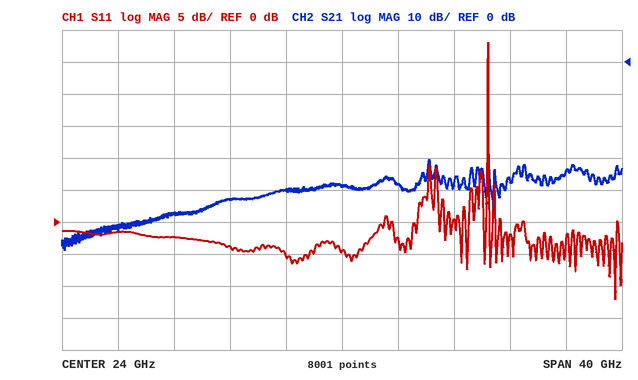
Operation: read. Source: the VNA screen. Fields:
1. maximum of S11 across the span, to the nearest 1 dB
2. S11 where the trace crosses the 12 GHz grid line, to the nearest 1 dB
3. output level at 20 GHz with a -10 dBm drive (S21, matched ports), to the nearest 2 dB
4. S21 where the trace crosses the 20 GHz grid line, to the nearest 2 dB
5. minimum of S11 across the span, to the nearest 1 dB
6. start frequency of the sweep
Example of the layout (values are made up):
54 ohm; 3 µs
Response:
28 dB; -2 dB; -50 dBm; -40 dB; -12 dB; 4 GHz
